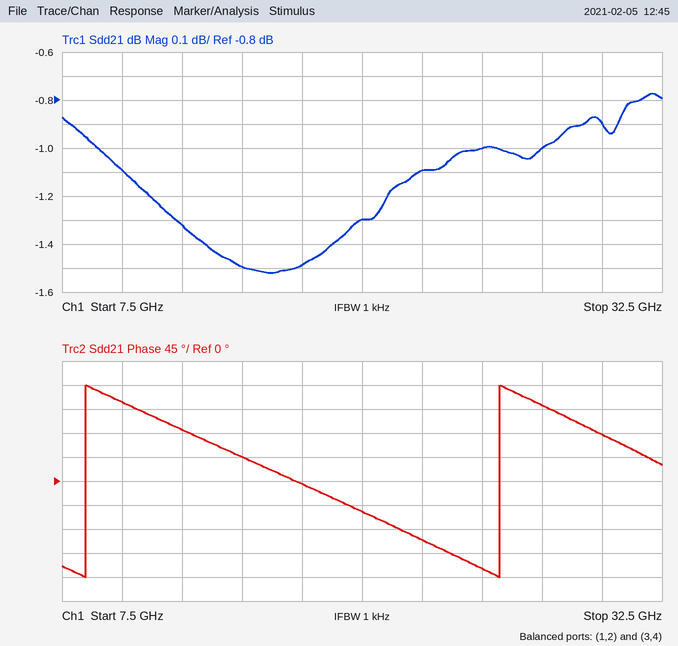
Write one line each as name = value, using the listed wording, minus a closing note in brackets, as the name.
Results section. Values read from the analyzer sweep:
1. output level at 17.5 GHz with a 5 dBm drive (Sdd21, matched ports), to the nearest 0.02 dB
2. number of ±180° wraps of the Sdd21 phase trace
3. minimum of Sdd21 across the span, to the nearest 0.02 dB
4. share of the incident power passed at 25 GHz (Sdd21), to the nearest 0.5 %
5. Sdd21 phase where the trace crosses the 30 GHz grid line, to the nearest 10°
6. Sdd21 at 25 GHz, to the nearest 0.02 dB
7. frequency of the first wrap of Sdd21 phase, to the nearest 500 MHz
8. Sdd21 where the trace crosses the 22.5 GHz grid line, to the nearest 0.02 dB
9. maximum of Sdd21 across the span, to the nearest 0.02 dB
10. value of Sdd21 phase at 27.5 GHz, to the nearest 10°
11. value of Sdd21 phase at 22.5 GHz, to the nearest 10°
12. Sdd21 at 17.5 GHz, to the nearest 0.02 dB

output level at 17.5 GHz with a 5 dBm drive (Sdd21, matched ports), to the nearest 0.02 dB = 3.52 dBm
number of ±180° wraps of the Sdd21 phase trace = 2
minimum of Sdd21 across the span, to the nearest 0.02 dB = -1.52 dB
share of the incident power passed at 25 GHz (Sdd21), to the nearest 0.5 % = 79.5 %
Sdd21 phase where the trace crosses the 30 GHz grid line, to the nearest 10° = 90°
Sdd21 at 25 GHz, to the nearest 0.02 dB = -1.00 dB
frequency of the first wrap of Sdd21 phase, to the nearest 500 MHz = 8.5 GHz
Sdd21 where the trace crosses the 22.5 GHz grid line, to the nearest 0.02 dB = -1.10 dB
maximum of Sdd21 across the span, to the nearest 0.02 dB = -0.78 dB
value of Sdd21 phase at 27.5 GHz, to the nearest 10° = 140°
value of Sdd21 phase at 22.5 GHz, to the nearest 10° = -110°
Sdd21 at 17.5 GHz, to the nearest 0.02 dB = -1.48 dB
